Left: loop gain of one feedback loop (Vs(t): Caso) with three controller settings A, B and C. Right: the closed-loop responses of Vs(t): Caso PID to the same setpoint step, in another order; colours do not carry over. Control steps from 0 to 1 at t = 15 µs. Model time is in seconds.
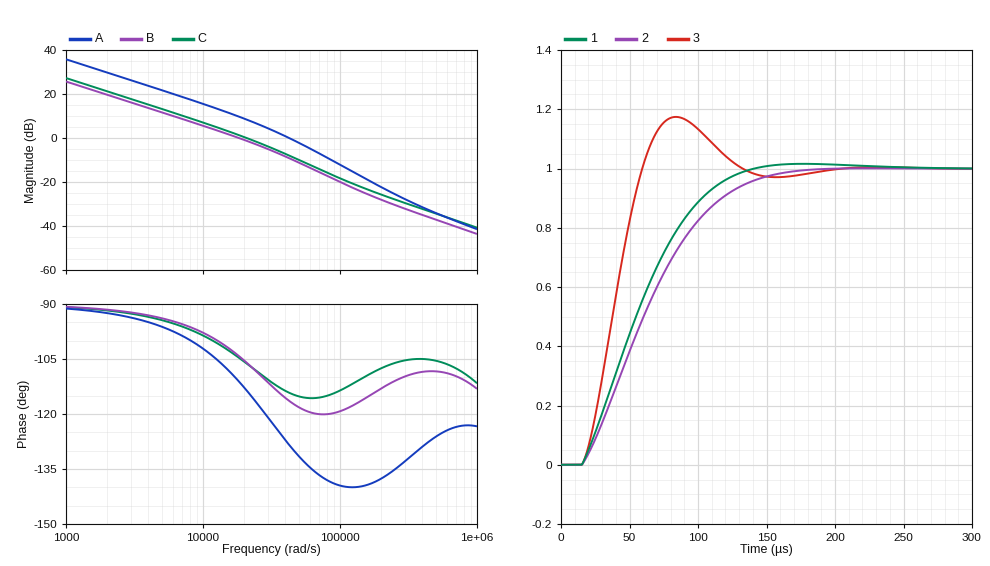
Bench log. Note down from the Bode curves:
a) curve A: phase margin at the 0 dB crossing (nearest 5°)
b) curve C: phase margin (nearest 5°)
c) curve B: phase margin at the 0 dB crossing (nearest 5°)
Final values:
50°
75°
75°
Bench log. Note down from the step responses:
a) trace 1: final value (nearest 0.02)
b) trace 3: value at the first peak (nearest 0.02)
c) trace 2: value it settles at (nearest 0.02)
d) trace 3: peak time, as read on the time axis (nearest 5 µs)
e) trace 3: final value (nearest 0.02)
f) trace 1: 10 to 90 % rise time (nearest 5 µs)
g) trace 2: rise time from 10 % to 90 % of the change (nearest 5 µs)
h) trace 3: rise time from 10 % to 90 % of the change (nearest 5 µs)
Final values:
1.00
1.18
1.00
85 µs
1.00
80 µs
90 µs
30 µs
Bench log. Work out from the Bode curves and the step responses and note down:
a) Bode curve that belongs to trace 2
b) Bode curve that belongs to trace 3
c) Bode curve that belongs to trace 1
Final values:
B
A
C
